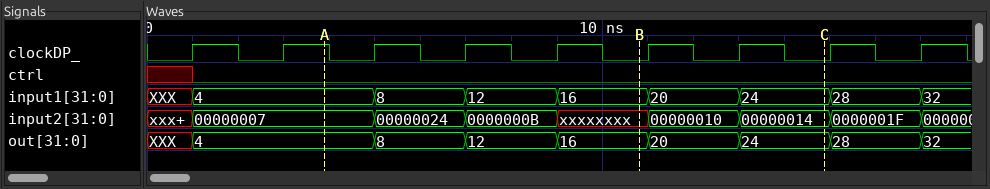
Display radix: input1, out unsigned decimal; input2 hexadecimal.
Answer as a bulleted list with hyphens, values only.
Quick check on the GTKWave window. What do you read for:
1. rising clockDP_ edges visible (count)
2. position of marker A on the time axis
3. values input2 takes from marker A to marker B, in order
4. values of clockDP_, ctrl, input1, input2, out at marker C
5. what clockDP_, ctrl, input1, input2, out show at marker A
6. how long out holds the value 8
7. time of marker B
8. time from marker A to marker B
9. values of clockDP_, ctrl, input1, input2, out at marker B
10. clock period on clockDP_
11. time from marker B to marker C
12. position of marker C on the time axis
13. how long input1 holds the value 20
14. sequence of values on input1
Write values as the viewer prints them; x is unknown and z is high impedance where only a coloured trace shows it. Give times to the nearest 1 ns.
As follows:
- 9
- 4 ns
- 00000007, 00000024, 0000000B, xxxxxxxx
- clockDP_=0, ctrl=0, input1=24, input2=00000014, out=24
- clockDP_=1, ctrl=0, input1=4, input2=00000007, out=4
- 2 ns
- 11 ns
- 7 ns
- clockDP_=0, ctrl=0, input1=16, input2=xxxxxxxx, out=16
- 2 ns
- 4 ns
- 15 ns
- 2 ns
- XXX, 4, 8, 12, 16, 20, 24, 28, 32
